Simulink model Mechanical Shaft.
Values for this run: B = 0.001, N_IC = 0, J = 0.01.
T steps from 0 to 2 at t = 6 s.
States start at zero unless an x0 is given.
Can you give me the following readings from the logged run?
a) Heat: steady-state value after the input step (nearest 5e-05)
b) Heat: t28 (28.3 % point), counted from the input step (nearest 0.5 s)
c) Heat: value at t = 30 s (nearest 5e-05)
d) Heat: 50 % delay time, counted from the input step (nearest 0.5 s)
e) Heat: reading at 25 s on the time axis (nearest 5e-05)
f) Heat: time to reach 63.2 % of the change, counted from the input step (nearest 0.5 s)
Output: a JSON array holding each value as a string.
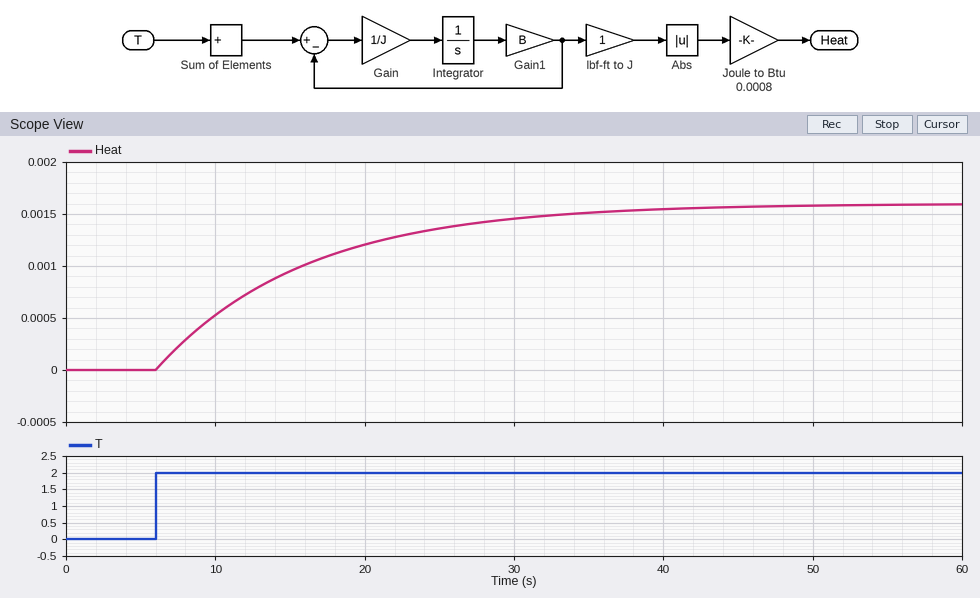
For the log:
["0.00160", "3.5 s", "0.00145", "7.0 s", "0.00135", "10.0 s"]
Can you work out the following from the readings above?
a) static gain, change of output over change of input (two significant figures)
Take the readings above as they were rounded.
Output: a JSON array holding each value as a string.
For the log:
["0.00080"]
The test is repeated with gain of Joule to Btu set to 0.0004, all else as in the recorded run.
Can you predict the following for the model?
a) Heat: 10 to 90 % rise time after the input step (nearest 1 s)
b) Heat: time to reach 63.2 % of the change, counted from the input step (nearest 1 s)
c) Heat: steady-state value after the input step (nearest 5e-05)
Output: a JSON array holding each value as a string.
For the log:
["22 s", "10 s", "0.00080"]
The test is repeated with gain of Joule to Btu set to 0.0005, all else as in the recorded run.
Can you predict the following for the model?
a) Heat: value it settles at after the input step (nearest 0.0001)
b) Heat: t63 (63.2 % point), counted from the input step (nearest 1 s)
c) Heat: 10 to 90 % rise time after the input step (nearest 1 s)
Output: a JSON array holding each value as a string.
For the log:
["0.0010", "10 s", "22 s"]
